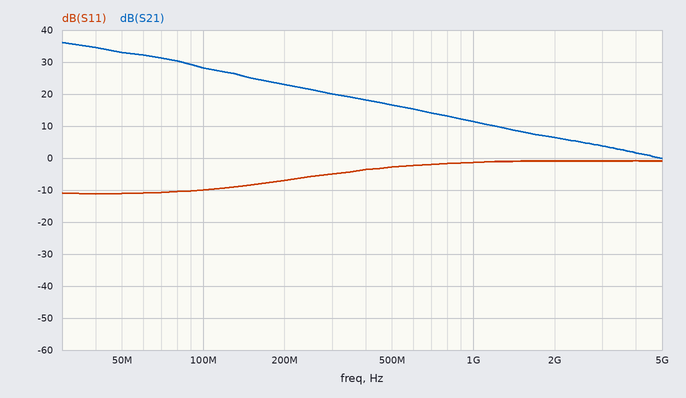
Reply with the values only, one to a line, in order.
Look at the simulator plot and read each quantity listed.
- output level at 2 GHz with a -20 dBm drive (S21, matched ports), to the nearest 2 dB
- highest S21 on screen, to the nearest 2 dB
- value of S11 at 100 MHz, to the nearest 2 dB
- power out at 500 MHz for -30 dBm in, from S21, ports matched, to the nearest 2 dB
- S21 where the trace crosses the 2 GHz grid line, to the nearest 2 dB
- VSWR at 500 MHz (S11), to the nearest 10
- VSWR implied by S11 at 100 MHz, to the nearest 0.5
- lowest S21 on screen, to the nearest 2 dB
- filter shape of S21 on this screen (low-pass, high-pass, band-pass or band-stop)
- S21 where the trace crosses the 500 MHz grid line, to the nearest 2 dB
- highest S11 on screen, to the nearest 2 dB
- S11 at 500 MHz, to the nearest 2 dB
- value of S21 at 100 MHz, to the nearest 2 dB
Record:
-14 dBm
36 dB
-10 dB
-14 dBm
6 dB
10
2.0
0 dB
low-pass
16 dB
0 dB
-2 dB
28 dB
